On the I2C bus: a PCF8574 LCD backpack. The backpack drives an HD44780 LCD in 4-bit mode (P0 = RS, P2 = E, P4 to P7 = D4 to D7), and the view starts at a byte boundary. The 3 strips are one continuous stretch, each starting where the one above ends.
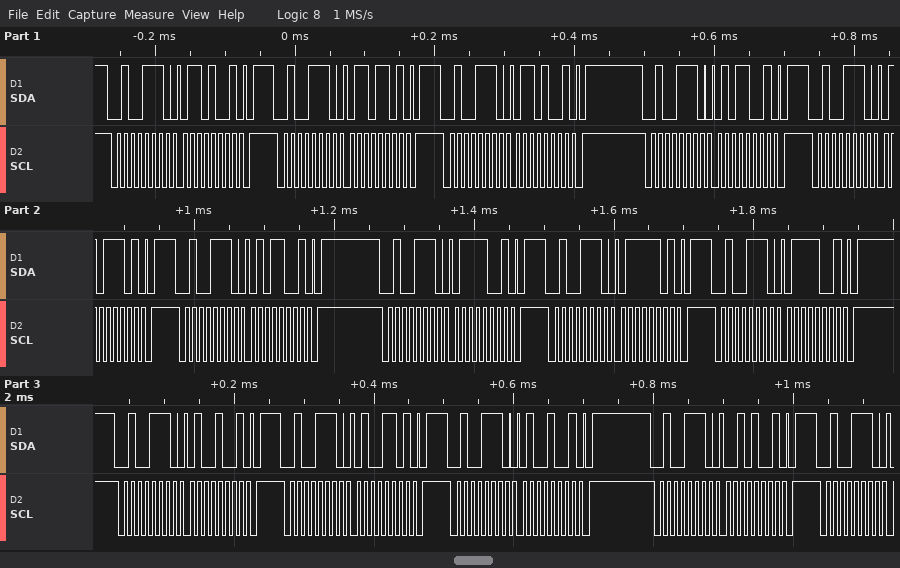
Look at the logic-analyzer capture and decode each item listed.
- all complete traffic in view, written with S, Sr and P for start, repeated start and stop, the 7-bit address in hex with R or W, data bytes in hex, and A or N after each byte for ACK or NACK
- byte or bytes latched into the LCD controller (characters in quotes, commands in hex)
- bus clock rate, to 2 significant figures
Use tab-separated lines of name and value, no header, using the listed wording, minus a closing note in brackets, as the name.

all complete traffic in view, written with S, Sr and P for start, repeated start and stop, the 7-bit address in hex with R or W, data bytes in hex, and A or N after each byte for ACK or NACK	S 27W A 69 A P S 27W A 6D A P S 27W A 69 A P S 27W A 59 A P S 27W A 5D A P S 27W A 59 A P S 27W A 79 A P S 27W A 7D A P S 27W A 79 A P S 27W A 49 A P S 27W A 4D A P S 27W A 49 A P S 27W A 29 A P S 27W A
byte or bytes latched into the LCD controller	'e' 't'
bus clock rate, to 2 significant figures	100 kHz
